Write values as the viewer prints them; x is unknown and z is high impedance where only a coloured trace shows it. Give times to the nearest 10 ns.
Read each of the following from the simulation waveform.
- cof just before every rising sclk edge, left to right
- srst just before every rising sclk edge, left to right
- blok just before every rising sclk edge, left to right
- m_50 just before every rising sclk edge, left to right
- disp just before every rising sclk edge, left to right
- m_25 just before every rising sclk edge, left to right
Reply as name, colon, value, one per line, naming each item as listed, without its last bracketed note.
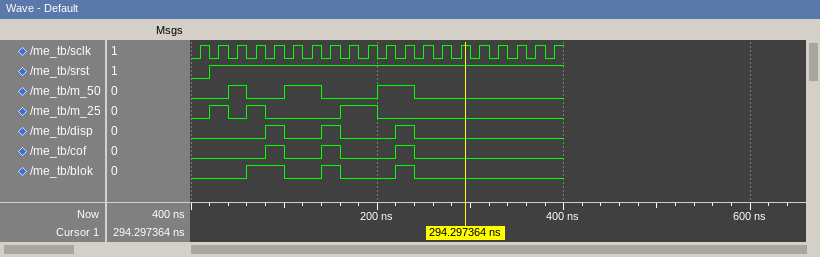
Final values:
cof just before every rising sclk edge, left to right: 0 0 0 0 1 0 0 1 0 0 0 1 0 0 0 0 0 0 0 0
srst just before every rising sclk edge, left to right: 0 1 1 1 1 1 1 1 1 1 1 1 1 1 1 1 1 1 1 1
blok just before every rising sclk edge, left to right: 0 0 0 1 1 0 0 1 0 0 0 1 0 0 0 0 0 0 0 0
m_50 just before every rising sclk edge, left to right: 0 0 1 0 0 1 1 0 0 0 1 1 0 0 0 0 0 0 0 0
disp just before every rising sclk edge, left to right: 0 0 0 0 1 0 0 1 0 0 0 1 0 0 0 0 0 0 0 0
m_25 just before every rising sclk edge, left to right: 0 1 0 1 0 0 0 0 1 1 0 0 0 0 0 0 0 0 0 0
